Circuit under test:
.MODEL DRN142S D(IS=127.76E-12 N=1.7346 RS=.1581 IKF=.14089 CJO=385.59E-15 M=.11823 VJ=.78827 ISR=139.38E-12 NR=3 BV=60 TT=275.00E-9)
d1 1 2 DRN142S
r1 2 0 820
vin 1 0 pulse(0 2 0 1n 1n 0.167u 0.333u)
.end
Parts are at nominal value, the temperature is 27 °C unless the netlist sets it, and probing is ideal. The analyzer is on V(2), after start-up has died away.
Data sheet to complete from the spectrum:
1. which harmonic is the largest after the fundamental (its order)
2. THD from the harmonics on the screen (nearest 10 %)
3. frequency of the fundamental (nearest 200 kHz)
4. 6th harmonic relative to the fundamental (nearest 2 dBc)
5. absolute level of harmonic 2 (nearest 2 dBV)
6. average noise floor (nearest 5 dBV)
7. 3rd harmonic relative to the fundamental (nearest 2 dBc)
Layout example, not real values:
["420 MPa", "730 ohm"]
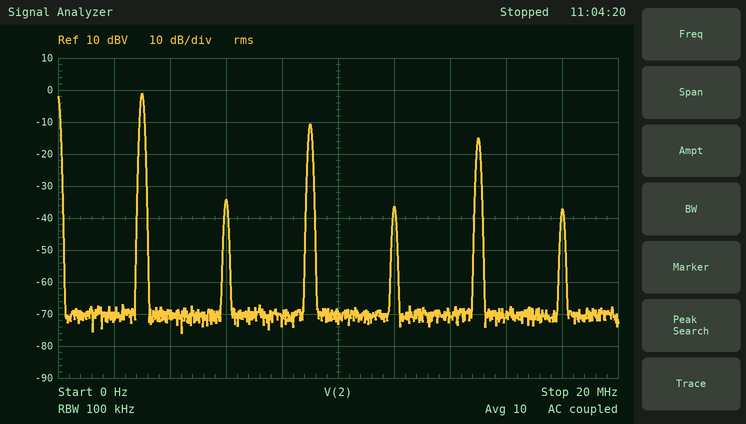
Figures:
["3", "40 %", "3.0 MHz", "-36 dBc", "-34 dBV", "-70 dBV", "-10 dBc"]
